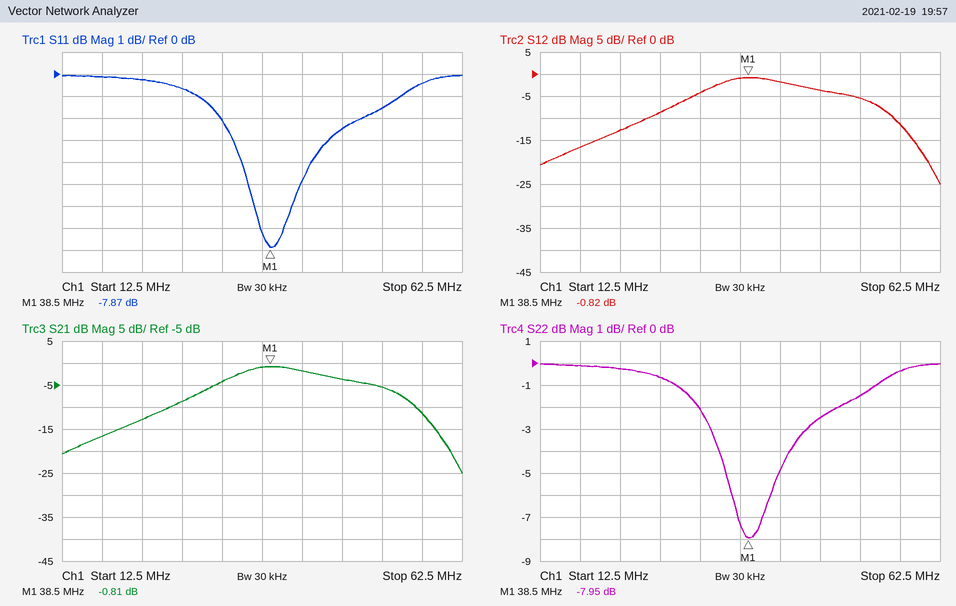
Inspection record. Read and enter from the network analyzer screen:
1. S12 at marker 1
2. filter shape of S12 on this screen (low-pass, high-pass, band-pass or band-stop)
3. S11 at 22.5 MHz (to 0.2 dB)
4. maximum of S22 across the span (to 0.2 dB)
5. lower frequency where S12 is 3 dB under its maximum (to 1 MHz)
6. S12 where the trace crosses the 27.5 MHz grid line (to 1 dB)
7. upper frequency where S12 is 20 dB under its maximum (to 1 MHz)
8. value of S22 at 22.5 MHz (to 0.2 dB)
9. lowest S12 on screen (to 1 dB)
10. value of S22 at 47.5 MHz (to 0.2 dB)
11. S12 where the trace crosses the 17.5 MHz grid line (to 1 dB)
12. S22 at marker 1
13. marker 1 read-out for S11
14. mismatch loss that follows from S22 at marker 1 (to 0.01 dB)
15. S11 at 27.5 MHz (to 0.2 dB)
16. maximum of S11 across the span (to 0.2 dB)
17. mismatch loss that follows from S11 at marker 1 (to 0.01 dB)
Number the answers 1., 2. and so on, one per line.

1. -0.82 dB
2. band-pass
3. -0.2 dB
4. 0.0 dB
5. 33 MHz
6. -9 dB
7. 61 MHz
8. -0.2 dB
9. -25 dB
10. -2.4 dB
11. -17 dB
12. -7.95 dB
13. -7.87 dB
14. 0.76 dB
15. -0.6 dB
16. 0.0 dB
17. 0.77 dB
